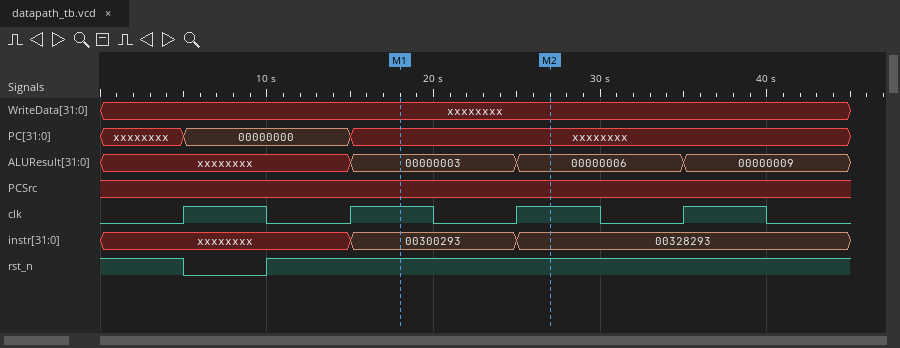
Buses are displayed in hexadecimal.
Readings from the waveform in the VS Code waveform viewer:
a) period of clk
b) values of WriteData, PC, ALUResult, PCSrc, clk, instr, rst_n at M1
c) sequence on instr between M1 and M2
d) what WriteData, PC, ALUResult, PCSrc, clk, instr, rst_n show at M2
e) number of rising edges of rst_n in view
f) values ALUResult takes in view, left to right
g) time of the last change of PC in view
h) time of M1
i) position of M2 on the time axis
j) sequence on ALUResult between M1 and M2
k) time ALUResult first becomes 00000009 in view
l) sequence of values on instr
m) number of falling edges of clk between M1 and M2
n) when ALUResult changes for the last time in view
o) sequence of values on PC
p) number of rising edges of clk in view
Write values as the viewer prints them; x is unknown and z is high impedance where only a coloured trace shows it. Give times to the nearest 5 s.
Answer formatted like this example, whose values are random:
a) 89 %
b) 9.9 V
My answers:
a) 10 s
b) WriteData=xxxxxxxx, PC=xxxxxxxx, ALUResult=00000003, PCSrc=x, clk=1, instr=00300293, rst_n=1
c) 00300293, 00328293
d) WriteData=xxxxxxxx, PC=xxxxxxxx, ALUResult=00000006, PCSrc=x, clk=1, instr=00328293, rst_n=1
e) 1
f) xxxxxxxx, 00000003, 00000006, 00000009
g) 15 s
h) 20 s
i) 25 s
j) 00000003, 00000006
k) 35 s
l) xxxxxxxx, 00300293, 00328293
m) 1
n) 35 s
o) xxxxxxxx, 00000000, xxxxxxxx
p) 4
